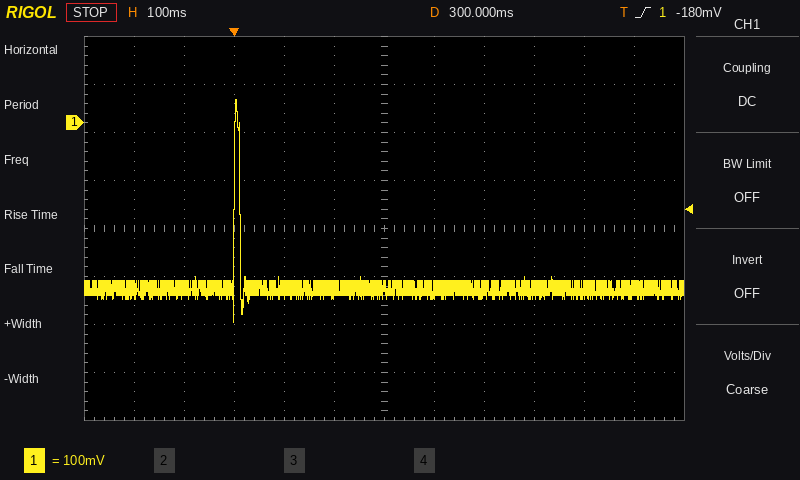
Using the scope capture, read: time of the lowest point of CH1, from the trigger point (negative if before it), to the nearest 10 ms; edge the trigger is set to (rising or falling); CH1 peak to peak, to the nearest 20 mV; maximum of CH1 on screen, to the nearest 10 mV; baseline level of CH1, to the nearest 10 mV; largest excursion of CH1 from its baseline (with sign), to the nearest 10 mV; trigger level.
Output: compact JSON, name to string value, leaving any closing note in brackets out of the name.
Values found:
{"time of the lowest point of CH1, from the trigger point (negative if before it), to the nearest 10 ms": "0 ms", "edge the trigger is set to": "rising", "CH1 peak to peak, to the nearest 20 mV": "460 mV", "maximum of CH1 on screen, to the nearest 10 mV": "50 mV", "baseline level of CH1, to the nearest 10 mV": "-340 mV", "largest excursion of CH1 from its baseline (with sign), to the nearest 10 mV": "+390 mV", "trigger level": "-180 mV"}
